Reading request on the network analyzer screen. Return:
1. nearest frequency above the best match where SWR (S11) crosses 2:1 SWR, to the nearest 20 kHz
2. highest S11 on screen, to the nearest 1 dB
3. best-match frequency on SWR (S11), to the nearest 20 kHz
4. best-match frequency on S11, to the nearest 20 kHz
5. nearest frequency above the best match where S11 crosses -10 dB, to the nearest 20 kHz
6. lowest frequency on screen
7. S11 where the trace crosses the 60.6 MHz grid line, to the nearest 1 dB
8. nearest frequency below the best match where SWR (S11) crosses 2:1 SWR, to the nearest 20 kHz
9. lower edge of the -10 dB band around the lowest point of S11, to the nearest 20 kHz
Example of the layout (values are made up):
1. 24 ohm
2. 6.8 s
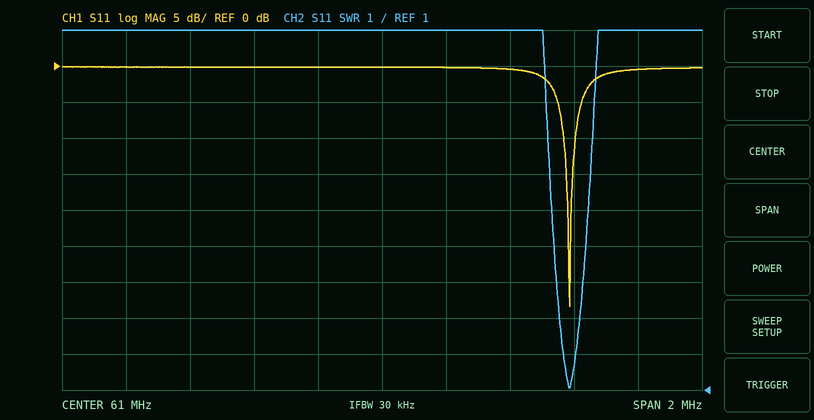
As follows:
1. 61.60 MHz
2. 0 dB
3. 61.58 MHz
4. 61.58 MHz
5. 61.60 MHz
6. 60 MHz
7. 0 dB
8. 61.56 MHz
9. 61.56 MHz
